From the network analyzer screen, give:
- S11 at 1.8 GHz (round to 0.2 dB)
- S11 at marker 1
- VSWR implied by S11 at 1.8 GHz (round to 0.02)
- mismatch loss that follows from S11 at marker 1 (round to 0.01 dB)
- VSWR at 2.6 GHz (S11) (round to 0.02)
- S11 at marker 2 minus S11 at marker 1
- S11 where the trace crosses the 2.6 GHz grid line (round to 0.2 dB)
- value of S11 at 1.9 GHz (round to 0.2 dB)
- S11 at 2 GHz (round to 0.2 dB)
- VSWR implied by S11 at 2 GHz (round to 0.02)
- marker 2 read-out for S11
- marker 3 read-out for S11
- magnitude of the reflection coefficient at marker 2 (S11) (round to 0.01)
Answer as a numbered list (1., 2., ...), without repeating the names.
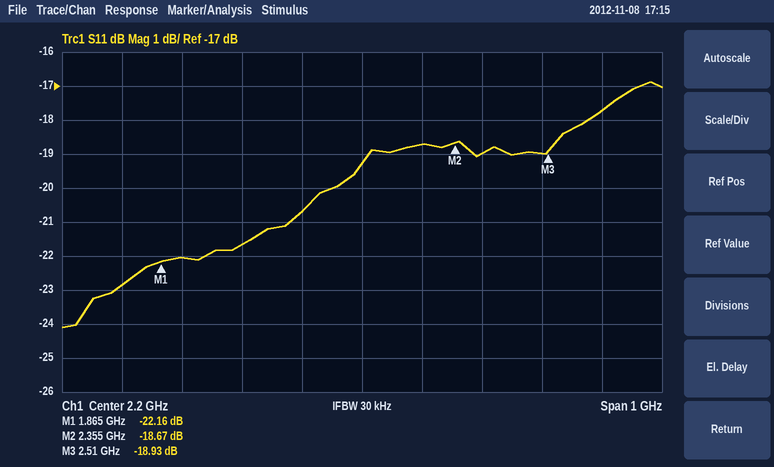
1. -22.8 dB
2. -22.16 dB
3. 1.16
4. 0.03 dB
5. 1.30
6. 3.49 dB
7. -17.8 dB
8. -22.0 dB
9. -21.6 dB
10. 1.18
11. -18.67 dB
12. -18.93 dB
13. 0.12
